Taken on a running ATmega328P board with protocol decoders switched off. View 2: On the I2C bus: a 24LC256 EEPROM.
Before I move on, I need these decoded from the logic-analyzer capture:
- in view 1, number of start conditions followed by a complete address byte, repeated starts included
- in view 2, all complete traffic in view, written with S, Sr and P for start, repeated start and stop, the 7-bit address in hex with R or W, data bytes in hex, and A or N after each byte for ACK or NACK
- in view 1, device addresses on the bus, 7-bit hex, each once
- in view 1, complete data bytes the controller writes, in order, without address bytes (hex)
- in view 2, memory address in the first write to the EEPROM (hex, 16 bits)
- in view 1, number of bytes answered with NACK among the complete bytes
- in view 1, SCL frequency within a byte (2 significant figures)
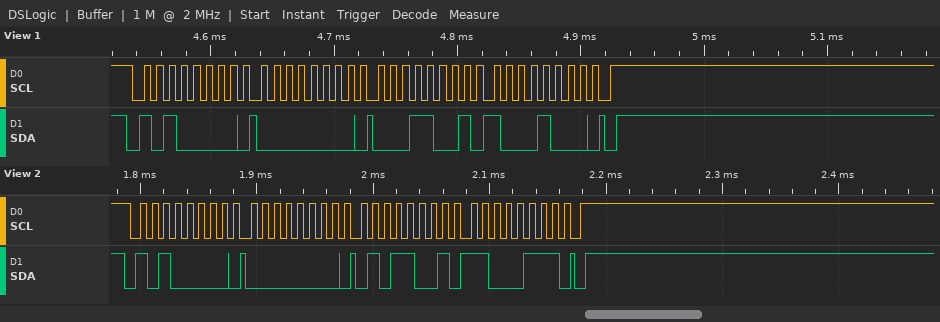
1
S 50W A 00 A 59 A C7 A P
0x50
00 19 88
0x0059
0
100 kHz
